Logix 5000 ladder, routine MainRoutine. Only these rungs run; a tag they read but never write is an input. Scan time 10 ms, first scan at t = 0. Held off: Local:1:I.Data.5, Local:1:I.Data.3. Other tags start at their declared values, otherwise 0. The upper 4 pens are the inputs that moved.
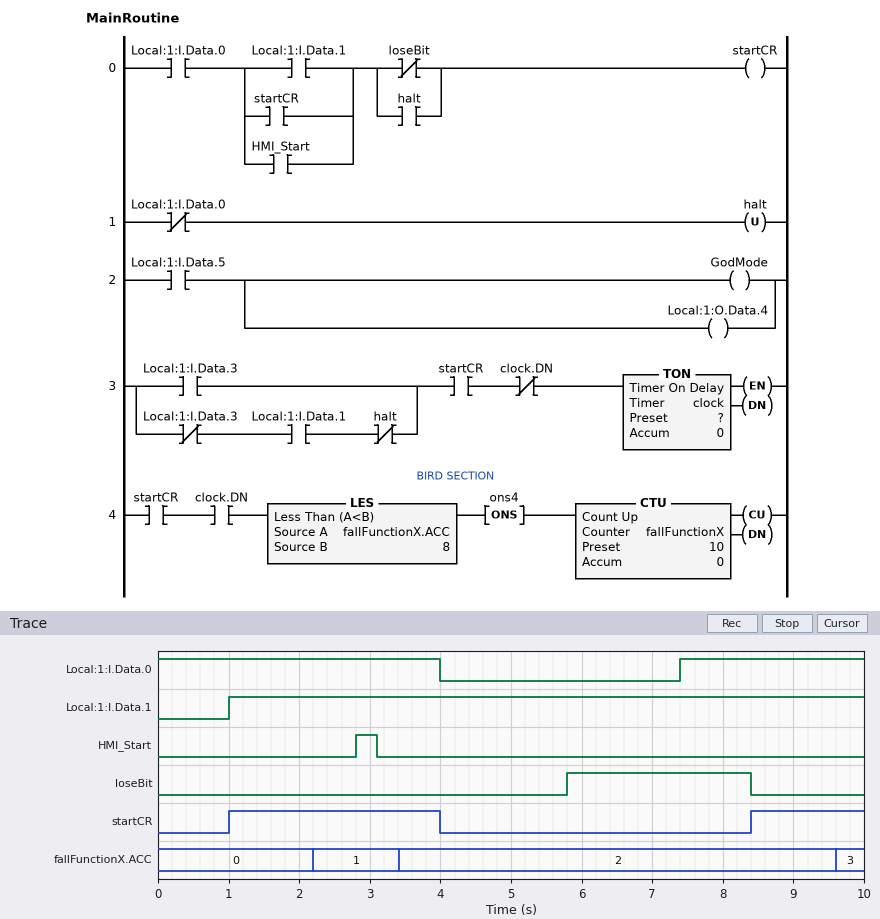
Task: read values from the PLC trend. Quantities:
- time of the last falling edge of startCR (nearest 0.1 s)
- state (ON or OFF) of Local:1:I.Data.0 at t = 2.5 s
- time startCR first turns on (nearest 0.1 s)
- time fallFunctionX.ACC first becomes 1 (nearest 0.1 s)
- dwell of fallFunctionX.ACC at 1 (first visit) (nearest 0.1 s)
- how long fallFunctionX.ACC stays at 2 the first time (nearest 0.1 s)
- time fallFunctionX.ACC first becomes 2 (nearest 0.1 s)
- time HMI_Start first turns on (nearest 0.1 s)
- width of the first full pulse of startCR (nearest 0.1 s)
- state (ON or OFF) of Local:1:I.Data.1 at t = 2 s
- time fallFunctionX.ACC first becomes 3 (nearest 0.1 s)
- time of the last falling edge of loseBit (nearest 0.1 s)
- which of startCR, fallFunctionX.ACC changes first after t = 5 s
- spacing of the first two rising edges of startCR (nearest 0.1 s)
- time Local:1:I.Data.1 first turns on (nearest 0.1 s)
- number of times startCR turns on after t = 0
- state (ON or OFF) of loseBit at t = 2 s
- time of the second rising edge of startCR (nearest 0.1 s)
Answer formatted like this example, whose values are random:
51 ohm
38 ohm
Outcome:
4.0 s
ON
1.0 s
2.2 s
1.2 s
6.2 s
3.4 s
2.8 s
3.0 s
ON
9.6 s
8.4 s
startCR
7.4 s
1.0 s
2
OFF
8.4 s
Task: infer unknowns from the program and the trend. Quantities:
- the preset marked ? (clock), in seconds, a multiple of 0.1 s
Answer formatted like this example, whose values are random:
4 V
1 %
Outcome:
1.2 s
